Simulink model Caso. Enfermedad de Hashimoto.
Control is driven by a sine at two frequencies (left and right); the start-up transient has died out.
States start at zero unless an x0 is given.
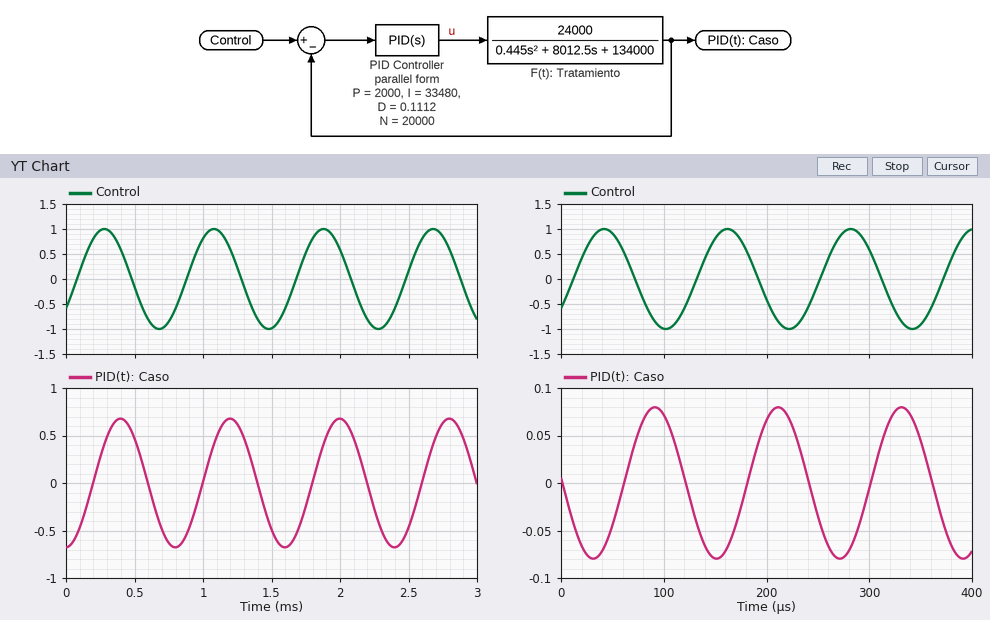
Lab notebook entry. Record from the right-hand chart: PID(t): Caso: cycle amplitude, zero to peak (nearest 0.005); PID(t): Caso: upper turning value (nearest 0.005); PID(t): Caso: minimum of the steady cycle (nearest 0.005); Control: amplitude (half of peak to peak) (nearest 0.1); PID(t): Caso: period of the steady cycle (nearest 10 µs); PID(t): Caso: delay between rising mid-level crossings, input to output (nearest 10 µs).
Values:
0.080
0.080
-0.080
1.0
120 µs
50 µs
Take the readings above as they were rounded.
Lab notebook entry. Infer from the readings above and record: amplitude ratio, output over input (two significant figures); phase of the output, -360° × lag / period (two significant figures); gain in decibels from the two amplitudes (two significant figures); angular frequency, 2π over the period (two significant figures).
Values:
0.080
-150°
-22 dB
0.052 rad/µs
